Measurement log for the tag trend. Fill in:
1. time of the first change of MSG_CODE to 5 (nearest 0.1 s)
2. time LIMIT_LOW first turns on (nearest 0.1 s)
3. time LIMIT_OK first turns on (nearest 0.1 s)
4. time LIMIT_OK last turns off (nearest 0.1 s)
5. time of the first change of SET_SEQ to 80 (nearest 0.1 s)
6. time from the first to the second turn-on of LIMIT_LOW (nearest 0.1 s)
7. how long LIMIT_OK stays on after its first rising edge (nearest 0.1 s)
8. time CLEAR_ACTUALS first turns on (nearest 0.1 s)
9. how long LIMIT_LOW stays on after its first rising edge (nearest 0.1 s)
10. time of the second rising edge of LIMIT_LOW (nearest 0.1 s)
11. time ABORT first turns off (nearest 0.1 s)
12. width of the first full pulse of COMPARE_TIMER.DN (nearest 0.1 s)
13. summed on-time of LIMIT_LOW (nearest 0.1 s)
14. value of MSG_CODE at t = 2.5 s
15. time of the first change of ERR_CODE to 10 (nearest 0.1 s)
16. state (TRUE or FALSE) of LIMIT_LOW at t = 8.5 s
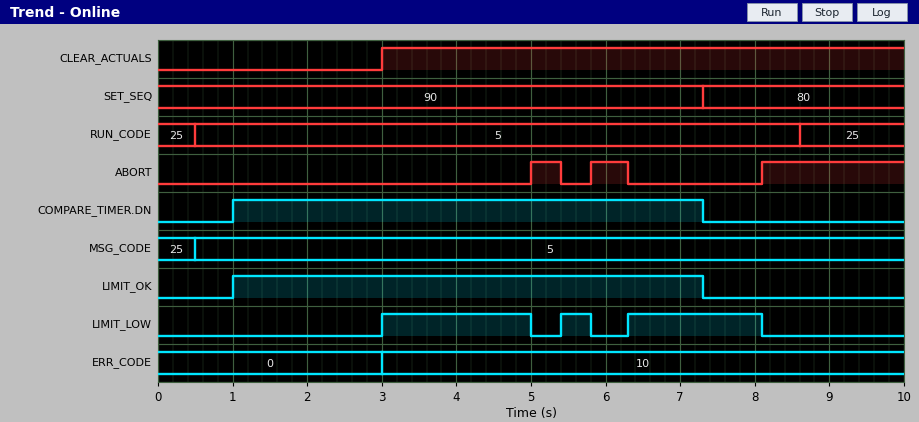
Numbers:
0.5 s
3.0 s
1.0 s
7.3 s
7.3 s
2.4 s
6.3 s
3.0 s
2.0 s
5.4 s
5.4 s
6.3 s
4.2 s
5
3.0 s
FALSE
